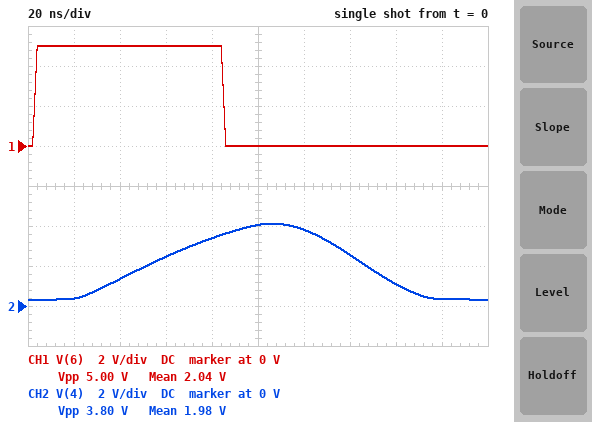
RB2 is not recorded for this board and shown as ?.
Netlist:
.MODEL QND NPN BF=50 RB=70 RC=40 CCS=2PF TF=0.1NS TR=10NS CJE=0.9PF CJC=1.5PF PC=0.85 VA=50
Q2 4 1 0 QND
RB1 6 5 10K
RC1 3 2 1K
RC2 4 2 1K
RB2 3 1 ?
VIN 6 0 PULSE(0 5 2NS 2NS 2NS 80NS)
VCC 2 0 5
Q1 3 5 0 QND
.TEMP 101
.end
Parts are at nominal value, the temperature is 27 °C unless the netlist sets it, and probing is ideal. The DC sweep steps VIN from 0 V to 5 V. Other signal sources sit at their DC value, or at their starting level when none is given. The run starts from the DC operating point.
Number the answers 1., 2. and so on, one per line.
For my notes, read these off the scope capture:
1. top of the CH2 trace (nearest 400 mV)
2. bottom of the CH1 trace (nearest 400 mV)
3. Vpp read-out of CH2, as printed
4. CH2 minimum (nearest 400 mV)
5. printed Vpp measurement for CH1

1. 4.0 V
2. 0 V
3. 3.80 V
4. 400 mV
5. 5.00 V
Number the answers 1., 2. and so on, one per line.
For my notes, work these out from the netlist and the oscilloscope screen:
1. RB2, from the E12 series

1. 22 kΩ
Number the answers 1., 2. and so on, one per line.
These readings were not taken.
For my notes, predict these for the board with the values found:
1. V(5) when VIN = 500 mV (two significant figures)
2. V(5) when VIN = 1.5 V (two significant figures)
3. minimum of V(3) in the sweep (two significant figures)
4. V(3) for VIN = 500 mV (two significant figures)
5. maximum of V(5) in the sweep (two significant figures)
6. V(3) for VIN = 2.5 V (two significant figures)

1. 500 mV
2. 720 mV
3. 280 mV
4. 4.8 V
5. 750 mV
6. 320 mV
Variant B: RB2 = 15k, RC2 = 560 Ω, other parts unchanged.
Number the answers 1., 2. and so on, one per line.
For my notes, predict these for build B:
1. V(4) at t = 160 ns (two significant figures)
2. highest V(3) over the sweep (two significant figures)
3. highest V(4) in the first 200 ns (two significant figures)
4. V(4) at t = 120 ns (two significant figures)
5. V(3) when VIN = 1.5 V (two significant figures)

1. 1.0 V
2. 4.7 V
3. 4.9 V
4. 4.3 V
5. 1.1 V
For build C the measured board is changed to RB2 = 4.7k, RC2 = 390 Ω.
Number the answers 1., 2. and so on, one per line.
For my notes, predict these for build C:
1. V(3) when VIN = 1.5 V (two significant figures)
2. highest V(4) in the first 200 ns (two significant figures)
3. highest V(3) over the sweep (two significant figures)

1. 1.0 V
2. 5.0 V
3. 4.3 V
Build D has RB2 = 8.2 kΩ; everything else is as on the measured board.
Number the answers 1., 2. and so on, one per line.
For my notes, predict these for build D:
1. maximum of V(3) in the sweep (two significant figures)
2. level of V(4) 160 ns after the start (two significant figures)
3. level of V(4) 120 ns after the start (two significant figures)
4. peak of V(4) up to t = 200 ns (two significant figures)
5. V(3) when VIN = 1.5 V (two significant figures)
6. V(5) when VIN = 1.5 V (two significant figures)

1. 4.5 V
2. 280 mV
3. 3.5 V
4. 4.8 V
5. 1.0 V
6. 720 mV
